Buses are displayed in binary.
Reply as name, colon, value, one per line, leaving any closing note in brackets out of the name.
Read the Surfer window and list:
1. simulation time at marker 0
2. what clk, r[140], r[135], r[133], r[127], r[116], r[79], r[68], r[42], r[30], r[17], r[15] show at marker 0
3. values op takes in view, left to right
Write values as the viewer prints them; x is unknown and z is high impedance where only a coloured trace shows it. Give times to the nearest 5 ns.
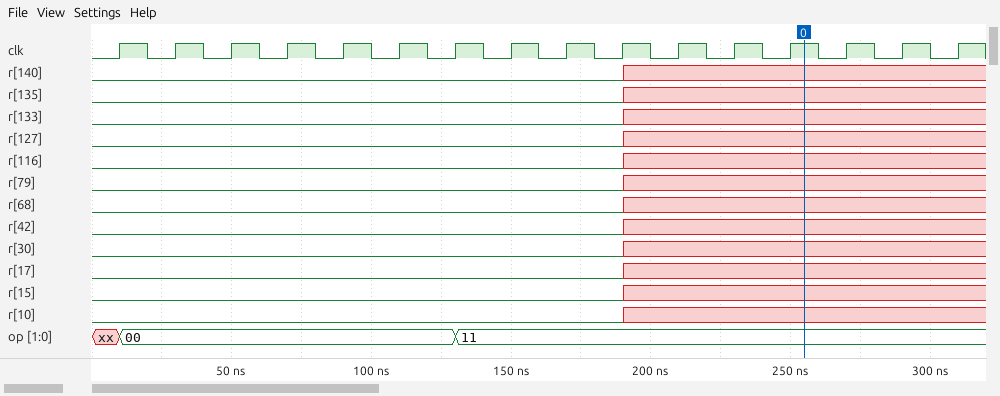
simulation time at marker 0: 255 ns
what clk, r[140], r[135], r[133], r[127], r[116], r[79], r[68], r[42], r[30], r[17], r[15] show at marker 0: clk=1, r[140]=x, r[135]=x, r[133]=x, r[127]=x, r[116]=x, r[79]=x, r[68]=x, r[42]=x, r[30]=x, r[17]=x, r[15]=x
values op takes in view, left to right: xx, 00, 11
